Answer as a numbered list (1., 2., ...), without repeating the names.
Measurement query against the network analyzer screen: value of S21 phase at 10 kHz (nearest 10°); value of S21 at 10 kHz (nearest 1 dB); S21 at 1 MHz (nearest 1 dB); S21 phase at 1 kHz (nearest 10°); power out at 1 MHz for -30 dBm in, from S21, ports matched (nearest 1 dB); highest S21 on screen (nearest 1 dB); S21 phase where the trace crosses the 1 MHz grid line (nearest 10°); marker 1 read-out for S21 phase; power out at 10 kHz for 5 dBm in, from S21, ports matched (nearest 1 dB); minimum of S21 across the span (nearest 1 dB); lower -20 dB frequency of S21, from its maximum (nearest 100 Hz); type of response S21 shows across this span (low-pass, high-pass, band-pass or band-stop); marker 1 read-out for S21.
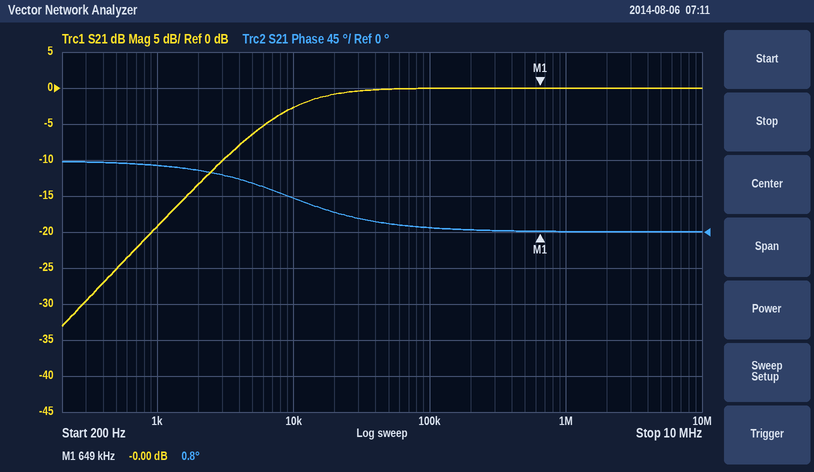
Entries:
1. 40°
2. -3 dB
3. 0 dB
4. 80°
5. -30 dBm
6. 0 dB
7. 0°
8. 0.8°
9. 2 dBm
10. -33 dB
11. 900 Hz
12. high-pass
13. -0.00 dB
